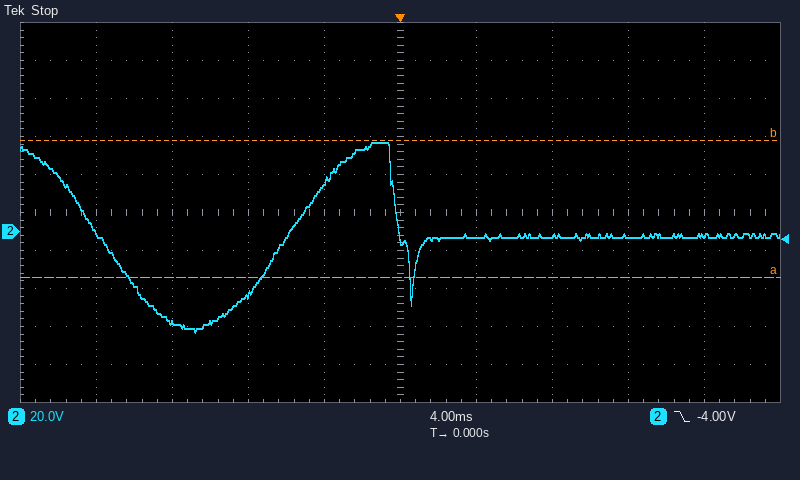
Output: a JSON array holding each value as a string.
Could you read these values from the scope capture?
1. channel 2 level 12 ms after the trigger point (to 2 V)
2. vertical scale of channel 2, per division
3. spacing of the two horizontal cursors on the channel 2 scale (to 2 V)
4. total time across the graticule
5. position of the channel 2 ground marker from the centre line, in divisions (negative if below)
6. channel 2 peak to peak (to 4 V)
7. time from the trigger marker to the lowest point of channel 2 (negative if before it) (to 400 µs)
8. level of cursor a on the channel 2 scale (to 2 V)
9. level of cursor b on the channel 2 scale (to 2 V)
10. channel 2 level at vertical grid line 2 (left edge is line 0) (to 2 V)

["-2 V", "20 V", "72 V", "40 ms", "-0.5 div", "100 V", "-10.8 ms", "-24 V", "48 V", "-48 V"]
